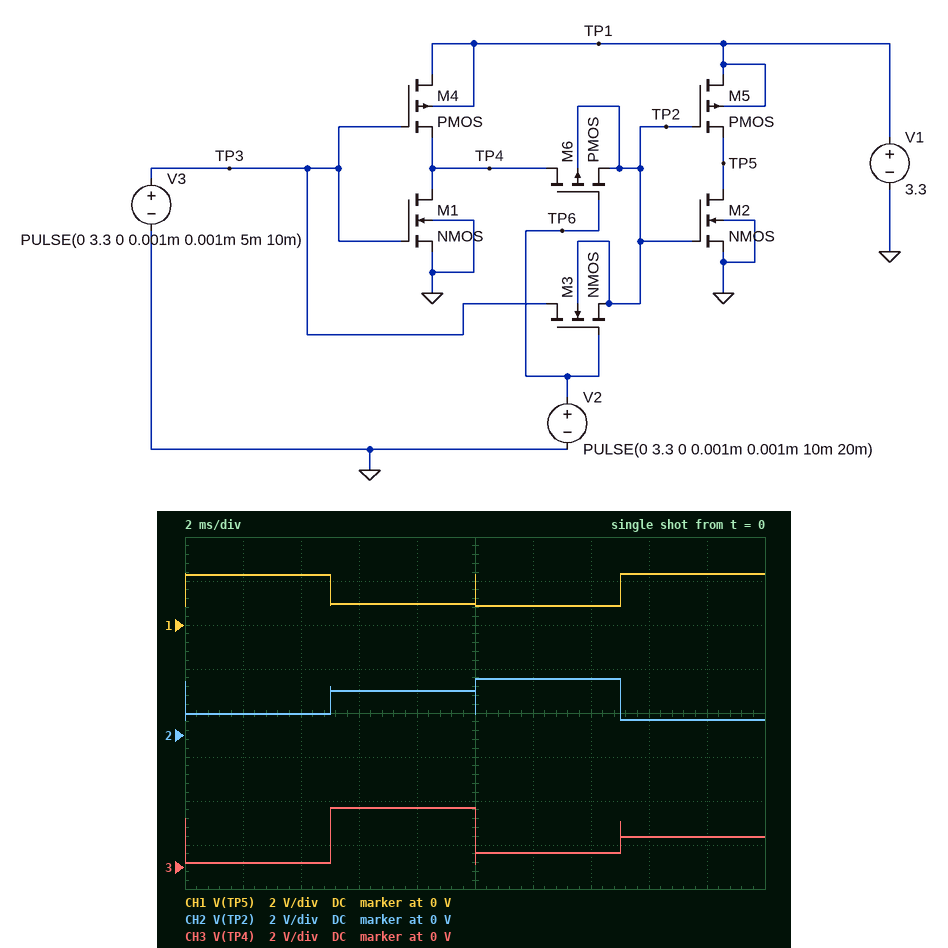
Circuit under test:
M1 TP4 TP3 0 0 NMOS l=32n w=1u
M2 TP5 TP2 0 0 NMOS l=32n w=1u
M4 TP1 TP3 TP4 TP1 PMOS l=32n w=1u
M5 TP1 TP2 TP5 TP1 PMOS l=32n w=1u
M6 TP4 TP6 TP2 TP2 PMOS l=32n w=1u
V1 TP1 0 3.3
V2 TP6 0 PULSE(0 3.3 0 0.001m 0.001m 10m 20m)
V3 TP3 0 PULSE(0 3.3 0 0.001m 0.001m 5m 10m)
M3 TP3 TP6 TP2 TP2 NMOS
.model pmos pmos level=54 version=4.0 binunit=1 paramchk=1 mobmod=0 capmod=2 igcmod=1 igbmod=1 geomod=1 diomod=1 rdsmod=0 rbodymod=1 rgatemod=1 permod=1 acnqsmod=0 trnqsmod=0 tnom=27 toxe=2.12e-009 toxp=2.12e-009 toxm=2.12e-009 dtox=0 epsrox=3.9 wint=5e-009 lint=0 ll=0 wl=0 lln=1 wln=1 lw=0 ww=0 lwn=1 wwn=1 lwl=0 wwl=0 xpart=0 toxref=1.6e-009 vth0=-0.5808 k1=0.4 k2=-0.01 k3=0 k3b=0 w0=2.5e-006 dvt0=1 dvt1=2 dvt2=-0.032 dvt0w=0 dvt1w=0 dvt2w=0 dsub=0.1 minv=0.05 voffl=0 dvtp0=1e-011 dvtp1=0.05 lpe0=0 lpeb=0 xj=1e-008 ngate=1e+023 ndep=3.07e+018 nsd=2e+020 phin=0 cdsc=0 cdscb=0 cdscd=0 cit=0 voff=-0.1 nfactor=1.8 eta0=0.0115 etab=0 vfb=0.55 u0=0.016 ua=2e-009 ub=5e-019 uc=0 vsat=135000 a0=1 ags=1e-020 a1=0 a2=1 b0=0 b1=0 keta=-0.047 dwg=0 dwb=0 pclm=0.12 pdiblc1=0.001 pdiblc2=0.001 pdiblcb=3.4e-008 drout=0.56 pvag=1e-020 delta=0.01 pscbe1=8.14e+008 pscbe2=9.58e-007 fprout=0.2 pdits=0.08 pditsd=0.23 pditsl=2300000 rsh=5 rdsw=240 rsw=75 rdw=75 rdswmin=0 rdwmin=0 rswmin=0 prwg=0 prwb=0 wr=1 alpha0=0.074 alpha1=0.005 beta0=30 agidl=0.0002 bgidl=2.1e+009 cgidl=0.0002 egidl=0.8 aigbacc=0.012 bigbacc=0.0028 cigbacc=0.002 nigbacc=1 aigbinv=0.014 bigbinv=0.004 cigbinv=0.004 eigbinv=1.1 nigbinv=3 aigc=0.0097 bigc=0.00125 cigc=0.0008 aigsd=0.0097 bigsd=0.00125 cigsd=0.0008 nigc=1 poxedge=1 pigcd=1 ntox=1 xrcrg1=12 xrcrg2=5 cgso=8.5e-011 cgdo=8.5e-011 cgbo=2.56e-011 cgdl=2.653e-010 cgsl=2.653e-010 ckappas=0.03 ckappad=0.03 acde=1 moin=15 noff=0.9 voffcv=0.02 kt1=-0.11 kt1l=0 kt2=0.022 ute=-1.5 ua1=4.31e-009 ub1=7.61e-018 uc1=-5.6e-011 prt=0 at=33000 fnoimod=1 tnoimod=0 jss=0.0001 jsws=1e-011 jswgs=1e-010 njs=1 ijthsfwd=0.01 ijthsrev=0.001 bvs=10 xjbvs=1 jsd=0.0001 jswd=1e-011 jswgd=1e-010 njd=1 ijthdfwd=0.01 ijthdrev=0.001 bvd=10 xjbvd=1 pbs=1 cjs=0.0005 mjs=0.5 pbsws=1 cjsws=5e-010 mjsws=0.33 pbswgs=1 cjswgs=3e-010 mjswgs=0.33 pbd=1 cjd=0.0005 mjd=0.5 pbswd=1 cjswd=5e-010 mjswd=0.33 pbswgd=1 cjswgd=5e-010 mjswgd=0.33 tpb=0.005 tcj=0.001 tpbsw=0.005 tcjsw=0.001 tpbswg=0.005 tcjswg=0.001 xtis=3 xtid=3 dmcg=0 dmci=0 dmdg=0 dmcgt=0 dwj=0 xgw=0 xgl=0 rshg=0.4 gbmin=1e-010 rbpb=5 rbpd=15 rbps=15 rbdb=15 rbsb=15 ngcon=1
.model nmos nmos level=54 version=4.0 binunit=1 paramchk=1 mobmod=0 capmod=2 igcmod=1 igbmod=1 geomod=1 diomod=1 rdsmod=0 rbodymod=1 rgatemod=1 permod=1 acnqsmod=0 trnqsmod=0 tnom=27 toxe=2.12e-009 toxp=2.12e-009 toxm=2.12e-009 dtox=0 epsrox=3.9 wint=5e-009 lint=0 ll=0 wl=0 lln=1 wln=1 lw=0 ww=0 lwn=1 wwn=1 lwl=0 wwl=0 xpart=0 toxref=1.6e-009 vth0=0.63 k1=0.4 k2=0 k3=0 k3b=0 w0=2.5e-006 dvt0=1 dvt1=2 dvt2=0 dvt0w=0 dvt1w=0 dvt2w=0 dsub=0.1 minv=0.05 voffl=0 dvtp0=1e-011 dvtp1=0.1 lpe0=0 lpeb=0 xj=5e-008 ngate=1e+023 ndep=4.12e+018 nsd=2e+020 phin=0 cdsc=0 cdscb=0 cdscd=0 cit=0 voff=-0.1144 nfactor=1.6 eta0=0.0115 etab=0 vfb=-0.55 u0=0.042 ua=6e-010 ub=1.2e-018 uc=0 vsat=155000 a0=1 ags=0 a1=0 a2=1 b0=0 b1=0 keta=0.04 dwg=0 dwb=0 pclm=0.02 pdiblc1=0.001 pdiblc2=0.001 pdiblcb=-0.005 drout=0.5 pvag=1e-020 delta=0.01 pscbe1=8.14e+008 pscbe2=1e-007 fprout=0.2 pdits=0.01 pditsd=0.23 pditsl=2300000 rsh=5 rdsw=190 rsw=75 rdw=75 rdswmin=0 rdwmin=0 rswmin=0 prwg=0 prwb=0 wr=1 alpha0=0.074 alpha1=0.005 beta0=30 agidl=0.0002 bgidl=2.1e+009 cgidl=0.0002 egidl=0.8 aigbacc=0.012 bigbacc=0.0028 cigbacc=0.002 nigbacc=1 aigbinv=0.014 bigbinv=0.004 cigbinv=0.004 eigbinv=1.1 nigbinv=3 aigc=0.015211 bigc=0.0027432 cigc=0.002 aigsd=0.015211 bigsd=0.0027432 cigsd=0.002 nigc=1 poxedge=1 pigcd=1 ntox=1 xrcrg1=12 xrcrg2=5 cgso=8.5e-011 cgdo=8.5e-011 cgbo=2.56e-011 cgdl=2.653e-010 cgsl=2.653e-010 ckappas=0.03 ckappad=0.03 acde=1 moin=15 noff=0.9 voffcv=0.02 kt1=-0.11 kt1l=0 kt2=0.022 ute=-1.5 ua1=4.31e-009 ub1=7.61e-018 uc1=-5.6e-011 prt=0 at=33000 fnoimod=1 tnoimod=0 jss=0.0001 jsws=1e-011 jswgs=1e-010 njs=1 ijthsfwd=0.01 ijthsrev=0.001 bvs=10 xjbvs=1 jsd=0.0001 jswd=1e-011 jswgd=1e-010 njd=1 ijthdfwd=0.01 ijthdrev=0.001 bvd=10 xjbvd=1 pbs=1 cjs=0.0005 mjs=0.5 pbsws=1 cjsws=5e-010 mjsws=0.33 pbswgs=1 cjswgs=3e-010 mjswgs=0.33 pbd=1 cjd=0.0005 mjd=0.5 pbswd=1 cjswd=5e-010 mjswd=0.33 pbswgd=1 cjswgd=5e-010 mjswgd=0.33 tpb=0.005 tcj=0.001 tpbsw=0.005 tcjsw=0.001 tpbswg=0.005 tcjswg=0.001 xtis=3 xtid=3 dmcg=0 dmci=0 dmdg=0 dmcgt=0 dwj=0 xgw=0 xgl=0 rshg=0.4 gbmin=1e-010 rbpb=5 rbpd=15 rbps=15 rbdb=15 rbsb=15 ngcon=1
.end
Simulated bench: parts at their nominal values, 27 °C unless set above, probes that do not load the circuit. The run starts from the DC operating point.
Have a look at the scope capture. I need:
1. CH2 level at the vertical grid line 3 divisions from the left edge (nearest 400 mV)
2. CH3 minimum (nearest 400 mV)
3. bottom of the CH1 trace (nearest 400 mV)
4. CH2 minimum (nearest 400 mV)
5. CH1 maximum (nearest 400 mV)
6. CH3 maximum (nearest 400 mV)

2.0 V
0 V
800 mV
800 mV
2.4 V
2.8 V
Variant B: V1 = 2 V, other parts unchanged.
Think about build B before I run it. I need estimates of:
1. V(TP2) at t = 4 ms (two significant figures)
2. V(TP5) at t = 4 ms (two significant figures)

900 mV
1.0 V
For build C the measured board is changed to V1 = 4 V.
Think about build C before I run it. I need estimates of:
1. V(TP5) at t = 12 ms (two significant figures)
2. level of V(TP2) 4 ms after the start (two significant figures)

1.4 V
2.6 V
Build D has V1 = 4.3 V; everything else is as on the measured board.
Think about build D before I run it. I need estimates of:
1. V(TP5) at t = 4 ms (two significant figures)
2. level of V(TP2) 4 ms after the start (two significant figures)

1.7 V
2.6 V
